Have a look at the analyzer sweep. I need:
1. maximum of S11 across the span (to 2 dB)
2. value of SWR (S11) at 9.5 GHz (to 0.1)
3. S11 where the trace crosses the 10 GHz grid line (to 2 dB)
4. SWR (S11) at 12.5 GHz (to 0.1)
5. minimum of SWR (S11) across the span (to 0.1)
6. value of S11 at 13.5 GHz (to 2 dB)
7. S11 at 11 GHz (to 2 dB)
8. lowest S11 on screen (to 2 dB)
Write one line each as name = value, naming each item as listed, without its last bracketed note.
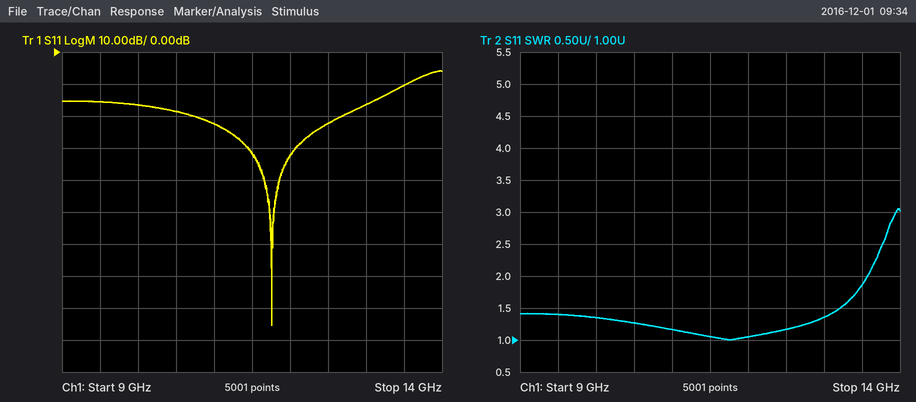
maximum of S11 across the span = -6 dB
value of SWR (S11) at 9.5 GHz = 1.4
S11 where the trace crosses the 10 GHz grid line = -16 dB
SWR (S11) at 12.5 GHz = 1.2
minimum of SWR (S11) across the span = 1.0
value of S11 at 13.5 GHz = -10 dB
S11 at 11 GHz = -22 dB
lowest S11 on screen = -86 dB
